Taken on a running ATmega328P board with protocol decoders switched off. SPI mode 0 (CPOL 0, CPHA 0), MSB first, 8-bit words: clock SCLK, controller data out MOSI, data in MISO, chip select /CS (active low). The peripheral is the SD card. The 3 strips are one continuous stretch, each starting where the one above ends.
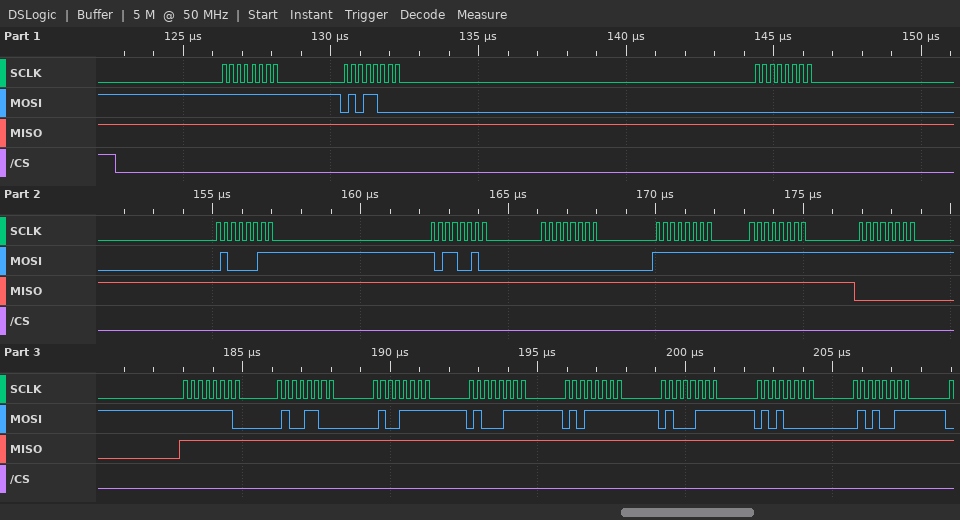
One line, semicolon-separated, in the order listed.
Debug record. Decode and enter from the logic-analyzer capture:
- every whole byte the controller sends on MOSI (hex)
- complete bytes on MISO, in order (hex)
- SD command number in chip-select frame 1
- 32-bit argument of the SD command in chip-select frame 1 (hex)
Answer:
0xFF 0x58 0x00 0x43 0xB2 0x00 0xFF 0xFF 0xFF 0xFE 0x4C 0x4F 0x47 0x5F 0x47 0x50 0x53; 0xFF 0xFF 0xFF 0xFF 0xFF 0xFF 0xFF 0xFF 0x00 0xFF 0xFF 0xFF 0xFF 0xFF 0xFF 0xFF 0xFF; CMD24; 0x0043B200
